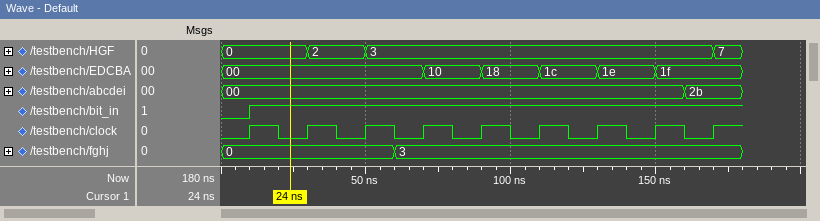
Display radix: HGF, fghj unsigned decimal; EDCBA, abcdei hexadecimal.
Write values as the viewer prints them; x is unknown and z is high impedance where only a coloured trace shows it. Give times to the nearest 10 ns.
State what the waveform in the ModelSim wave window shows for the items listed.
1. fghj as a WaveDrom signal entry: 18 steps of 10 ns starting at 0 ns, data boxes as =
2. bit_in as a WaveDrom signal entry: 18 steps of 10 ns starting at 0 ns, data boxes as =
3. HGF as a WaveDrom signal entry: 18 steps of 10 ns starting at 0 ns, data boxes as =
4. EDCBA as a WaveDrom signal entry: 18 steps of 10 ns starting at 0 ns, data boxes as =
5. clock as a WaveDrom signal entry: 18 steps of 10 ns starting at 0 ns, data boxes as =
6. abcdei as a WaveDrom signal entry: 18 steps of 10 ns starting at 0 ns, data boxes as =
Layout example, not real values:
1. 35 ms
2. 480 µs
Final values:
1. {name: 'fghj', wave: '=.....=...........', data: '0 3'}
2. {name: 'bit_in', wave: '01................'}
3. {name: 'HGF', wave: '=..=.=...........=', data: '0 2 3 7'}
4. {name: 'EDCBA', wave: '=......=.=.=.=.=..', data: '00 10 18 1c 1e 1f'}
5. {name: 'clock', wave: '010101010101010101'}
6. {name: 'abcdei', wave: '=...............=.', data: '00 2b'}
